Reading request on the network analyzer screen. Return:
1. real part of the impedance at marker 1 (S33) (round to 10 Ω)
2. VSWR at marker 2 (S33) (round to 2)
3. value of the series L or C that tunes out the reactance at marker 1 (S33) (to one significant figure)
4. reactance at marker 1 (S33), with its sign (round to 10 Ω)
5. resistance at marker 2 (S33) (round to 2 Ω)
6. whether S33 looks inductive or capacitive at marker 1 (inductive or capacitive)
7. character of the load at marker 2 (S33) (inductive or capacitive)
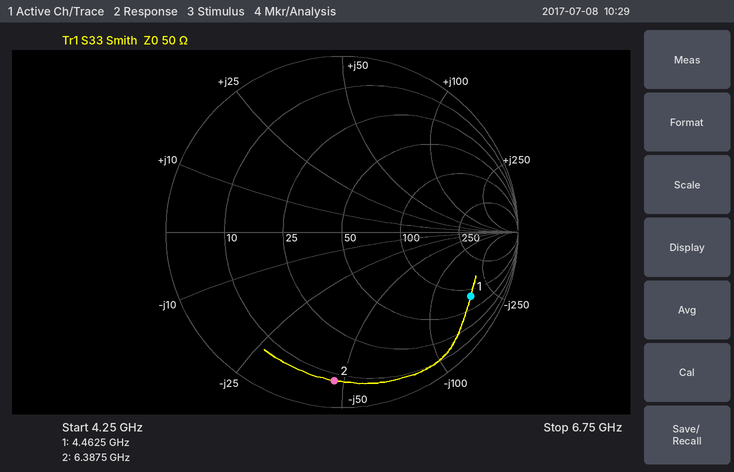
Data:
80 Ω
12
6 nH
-180 Ω
8 Ω
capacitive
capacitive
